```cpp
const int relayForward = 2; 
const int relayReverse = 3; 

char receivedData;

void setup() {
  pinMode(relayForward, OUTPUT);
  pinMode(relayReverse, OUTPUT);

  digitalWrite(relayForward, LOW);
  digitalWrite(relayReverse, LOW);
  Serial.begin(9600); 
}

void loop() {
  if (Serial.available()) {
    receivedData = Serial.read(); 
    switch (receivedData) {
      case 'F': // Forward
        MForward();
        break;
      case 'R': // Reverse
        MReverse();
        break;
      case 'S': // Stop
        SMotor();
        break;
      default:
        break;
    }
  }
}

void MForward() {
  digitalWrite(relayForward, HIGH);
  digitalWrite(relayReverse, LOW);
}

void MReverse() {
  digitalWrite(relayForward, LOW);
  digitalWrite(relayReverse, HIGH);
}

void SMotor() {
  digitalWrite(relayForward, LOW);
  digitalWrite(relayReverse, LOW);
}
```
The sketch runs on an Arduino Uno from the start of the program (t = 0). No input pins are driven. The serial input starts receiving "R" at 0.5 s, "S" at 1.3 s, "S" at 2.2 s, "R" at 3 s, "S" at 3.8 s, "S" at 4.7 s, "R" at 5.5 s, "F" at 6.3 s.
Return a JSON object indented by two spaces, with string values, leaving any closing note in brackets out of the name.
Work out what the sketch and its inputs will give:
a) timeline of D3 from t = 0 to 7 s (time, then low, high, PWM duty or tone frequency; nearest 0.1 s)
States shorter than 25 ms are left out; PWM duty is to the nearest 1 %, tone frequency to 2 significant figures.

{
  "timeline of D3 from t = 0 to 7 s": "0 s low; 0.5 s high; 1.3 s low; 3 s high; 3.8 s low; 5.5 s high; 6.3 s low"
}
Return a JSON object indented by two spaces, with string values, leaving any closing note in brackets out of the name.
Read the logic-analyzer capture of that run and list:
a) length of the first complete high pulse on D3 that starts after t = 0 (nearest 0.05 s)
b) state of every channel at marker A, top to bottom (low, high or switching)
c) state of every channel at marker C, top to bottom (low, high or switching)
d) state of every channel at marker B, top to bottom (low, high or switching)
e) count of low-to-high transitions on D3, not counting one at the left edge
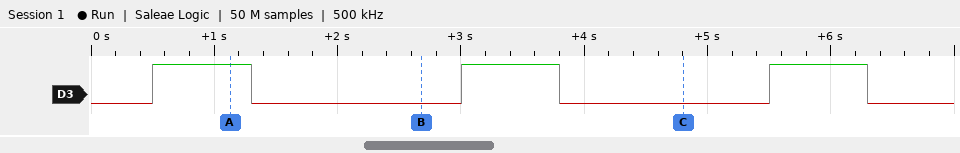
{
  "length of the first complete high pulse on D3 that starts after t = 0": "0.80 s",
  "state of every channel at marker A, top to bottom": "D3 high",
  "state of every channel at marker C, top to bottom": "D3 low",
  "state of every channel at marker B, top to bottom": "D3 low",
  "count of low-to-high transitions on D3, not counting one at the left edge": "3"
}
